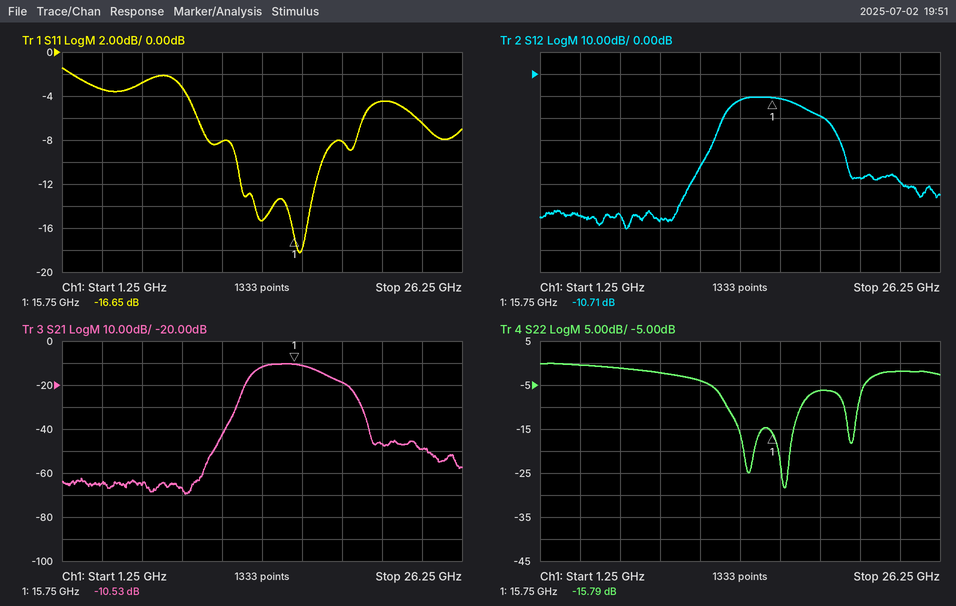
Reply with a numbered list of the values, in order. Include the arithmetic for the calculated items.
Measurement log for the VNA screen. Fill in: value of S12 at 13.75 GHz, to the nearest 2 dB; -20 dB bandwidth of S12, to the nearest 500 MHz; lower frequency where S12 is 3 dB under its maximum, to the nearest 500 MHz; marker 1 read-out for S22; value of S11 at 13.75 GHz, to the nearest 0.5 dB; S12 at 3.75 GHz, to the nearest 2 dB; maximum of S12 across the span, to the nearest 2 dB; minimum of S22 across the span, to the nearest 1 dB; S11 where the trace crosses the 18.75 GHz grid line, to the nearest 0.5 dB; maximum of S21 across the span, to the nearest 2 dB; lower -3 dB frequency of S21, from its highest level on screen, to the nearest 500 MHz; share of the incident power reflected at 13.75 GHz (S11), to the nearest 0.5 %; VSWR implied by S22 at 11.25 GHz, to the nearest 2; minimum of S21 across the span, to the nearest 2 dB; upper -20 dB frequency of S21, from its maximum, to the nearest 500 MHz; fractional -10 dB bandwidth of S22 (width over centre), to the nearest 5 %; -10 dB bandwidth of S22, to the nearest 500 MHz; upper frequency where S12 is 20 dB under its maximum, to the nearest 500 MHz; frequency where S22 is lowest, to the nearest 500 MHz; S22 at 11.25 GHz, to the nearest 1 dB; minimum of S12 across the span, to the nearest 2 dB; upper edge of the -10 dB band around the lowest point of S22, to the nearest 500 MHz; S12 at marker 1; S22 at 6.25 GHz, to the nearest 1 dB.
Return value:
1. -12 dB
2. 20.0 GHz − 12.0 GHz = 8.0 GHz
3. 13.5 GHz
4. -15.79 dB
5. -15.5 dB
6. -64 dB
7. -10 dB
8. -28 dB
9. -8.0 dB
10. -10 dB
11. 13.5 GHz
12. 10^(-15.5/10) ≈ 2.82 %, so 3.0 % to the nearest 0.5 %
13. |Γ| = 10^(-4/20) = 0.6310; VSWR = (1 + 0.6310)/(1 − 0.6310) ≈ 4
14. -70 dB
15. 20.0 GHz
16. 4.5 GHz / 15.25 GHz ≈ 30 %
17. 17.5 GHz − 13.0 GHz = 4.5 GHz
18. 20.0 GHz
19. 16.5 GHz
20. -4 dB
21. -70 dB
22. 17.5 GHz
23. -10.71 dB
24. -1 dB
